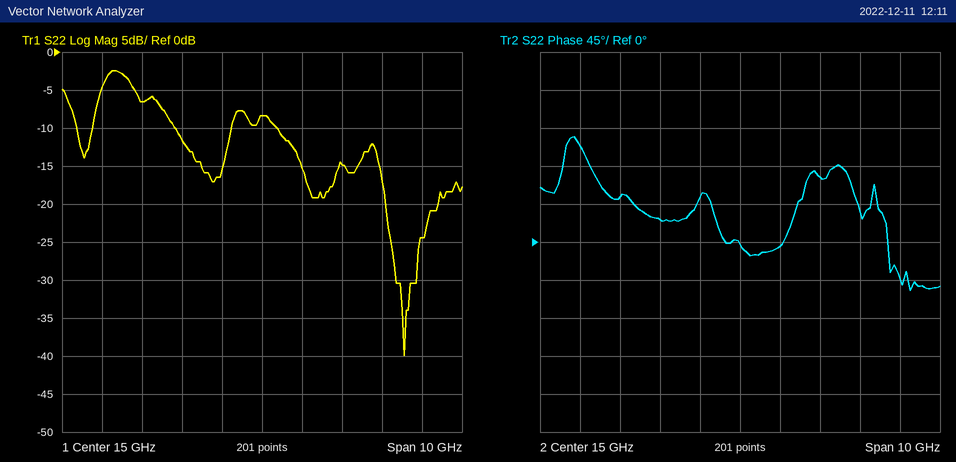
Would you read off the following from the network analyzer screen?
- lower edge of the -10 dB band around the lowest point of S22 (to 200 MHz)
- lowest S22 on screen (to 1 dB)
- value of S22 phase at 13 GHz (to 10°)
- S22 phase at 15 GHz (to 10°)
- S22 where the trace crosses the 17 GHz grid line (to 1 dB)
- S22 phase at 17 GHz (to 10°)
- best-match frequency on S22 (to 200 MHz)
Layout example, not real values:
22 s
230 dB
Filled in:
15.4 GHz
-40 dB
30°
0°
-15 dB
80°
18.6 GHz
